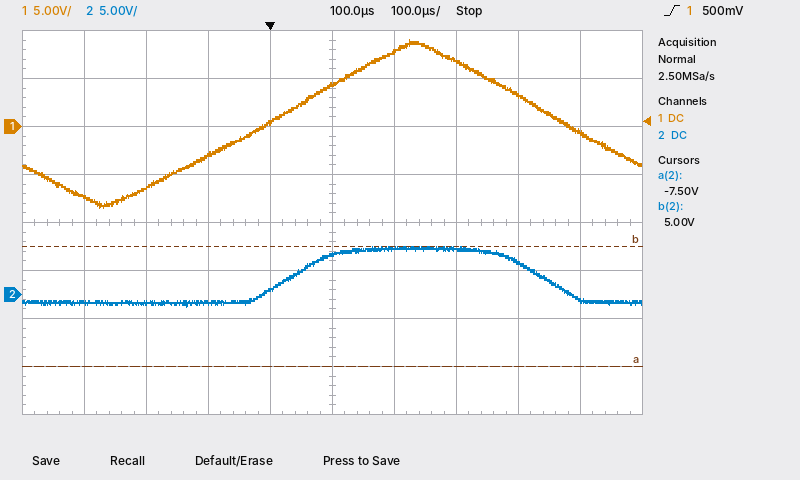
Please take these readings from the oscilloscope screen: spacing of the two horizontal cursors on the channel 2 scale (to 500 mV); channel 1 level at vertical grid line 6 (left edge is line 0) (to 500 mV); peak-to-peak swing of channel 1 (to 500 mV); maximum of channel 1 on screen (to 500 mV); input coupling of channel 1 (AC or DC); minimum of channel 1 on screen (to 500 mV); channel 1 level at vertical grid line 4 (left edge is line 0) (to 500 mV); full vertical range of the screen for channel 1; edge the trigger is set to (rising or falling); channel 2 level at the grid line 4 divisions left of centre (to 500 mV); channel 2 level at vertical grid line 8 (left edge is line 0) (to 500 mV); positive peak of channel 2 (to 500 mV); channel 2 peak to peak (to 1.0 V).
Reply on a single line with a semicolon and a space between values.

12.5 V; 8.0 V; 17.5 V; 9.0 V; DC; -8.5 V; 500 mV; 40 V; rising; -1.0 V; 3.5 V; 5.0 V; 6.0 V
